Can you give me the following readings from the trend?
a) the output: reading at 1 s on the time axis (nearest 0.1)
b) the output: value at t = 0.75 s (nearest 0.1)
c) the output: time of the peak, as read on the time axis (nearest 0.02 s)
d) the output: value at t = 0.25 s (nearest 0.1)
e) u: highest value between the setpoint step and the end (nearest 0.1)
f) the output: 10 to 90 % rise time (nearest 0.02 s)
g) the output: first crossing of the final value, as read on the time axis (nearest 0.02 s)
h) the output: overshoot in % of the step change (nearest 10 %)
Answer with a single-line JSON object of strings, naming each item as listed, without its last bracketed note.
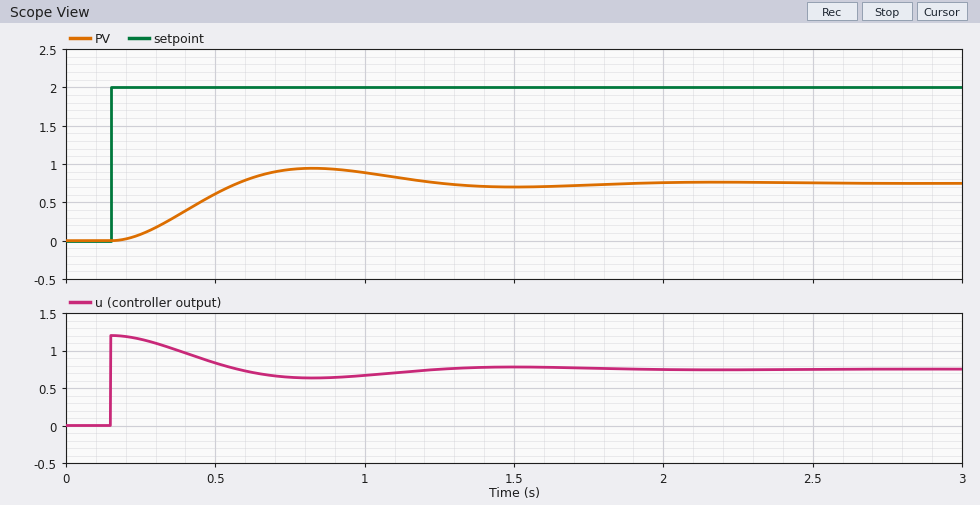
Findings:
{"the output: reading at 1 s on the time axis": "0.9", "the output: value at t = 0.75 s": "0.9", "the output: time of the peak, as read on the time axis": "0.82 s", "the output: value at t = 0.25 s": "0.1", "u: highest value between the setpoint step and the end": "1.2", "the output: 10 to 90 % rise time": "0.28 s", "the output: first crossing of the final value, as read on the time axis": "0.58 s", "the output: overshoot in % of the step change": "30 %"}
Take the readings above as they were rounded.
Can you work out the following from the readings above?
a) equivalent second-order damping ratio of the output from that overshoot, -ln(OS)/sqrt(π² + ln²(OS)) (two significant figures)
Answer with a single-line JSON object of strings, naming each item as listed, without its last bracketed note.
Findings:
{"equivalent second-order damping ratio of the output from that overshoot, -ln(OS)/sqrt(π² + ln²(OS))": "0.36"}
